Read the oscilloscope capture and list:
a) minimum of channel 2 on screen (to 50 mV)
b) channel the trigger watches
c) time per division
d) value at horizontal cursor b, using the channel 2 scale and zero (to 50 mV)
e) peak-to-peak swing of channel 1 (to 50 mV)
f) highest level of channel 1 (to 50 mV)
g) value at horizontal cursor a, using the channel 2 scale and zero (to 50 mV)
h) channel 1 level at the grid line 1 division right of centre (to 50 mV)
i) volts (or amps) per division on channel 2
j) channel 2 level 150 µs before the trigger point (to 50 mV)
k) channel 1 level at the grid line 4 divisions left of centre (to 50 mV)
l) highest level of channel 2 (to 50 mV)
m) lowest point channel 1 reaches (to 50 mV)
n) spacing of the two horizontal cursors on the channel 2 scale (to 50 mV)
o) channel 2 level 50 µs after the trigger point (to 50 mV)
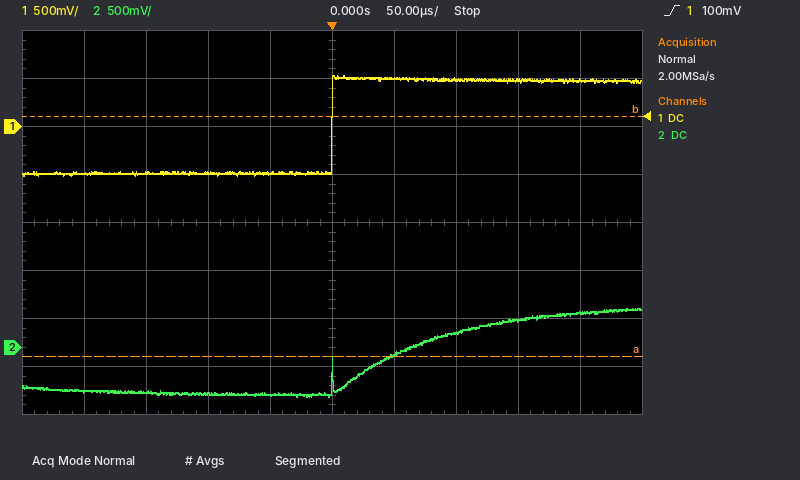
-500 mV
channel 1
50 µs
2.40 V
1.05 V
550 mV
-100 mV
500 mV
500 mV
-450 mV
-500 mV
400 mV
-500 mV
2.50 V
-50 mV
